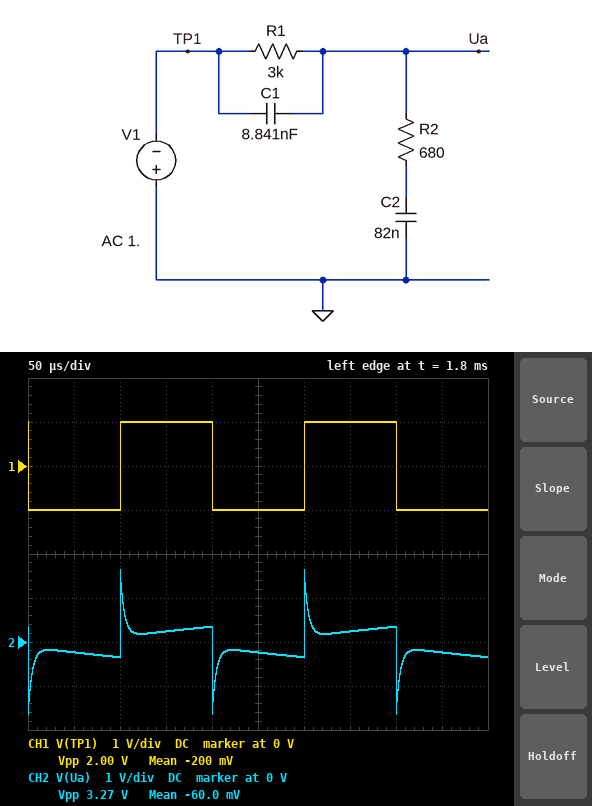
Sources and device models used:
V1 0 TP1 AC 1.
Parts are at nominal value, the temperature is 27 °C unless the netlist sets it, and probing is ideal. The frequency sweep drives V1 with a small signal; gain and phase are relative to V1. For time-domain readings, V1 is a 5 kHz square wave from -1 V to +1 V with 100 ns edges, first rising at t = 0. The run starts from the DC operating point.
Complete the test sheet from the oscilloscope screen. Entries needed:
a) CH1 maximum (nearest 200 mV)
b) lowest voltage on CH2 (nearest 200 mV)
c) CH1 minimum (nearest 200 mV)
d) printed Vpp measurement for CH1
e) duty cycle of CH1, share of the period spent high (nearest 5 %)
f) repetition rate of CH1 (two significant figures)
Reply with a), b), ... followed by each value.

a) 1.0 V
b) -1.6 V
c) -1.0 V
d) 2.00 V
e) 50 %
f) 5.0 kHz
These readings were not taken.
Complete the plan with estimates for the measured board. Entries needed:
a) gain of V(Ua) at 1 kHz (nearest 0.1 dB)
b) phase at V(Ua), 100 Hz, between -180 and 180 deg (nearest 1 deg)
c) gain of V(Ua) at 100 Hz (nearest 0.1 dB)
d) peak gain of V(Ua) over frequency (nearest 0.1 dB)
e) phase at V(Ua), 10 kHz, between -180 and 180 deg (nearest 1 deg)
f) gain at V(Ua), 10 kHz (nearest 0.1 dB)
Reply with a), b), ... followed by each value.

a) -6.5 dB
b) 171 deg
c) -0.2 dB
d) 0 dB
e) -150 deg
f) -9.5 dB
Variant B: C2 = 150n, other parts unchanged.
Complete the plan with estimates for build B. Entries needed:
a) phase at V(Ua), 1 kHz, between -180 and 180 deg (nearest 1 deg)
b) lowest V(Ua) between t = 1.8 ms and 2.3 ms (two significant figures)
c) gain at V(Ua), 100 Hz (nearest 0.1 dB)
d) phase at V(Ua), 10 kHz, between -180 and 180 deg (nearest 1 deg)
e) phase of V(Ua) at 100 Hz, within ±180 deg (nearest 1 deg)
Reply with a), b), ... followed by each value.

a) 146 deg
b) -1.7 V
c) -0.5 dB
d) -145 deg
e) 165 deg
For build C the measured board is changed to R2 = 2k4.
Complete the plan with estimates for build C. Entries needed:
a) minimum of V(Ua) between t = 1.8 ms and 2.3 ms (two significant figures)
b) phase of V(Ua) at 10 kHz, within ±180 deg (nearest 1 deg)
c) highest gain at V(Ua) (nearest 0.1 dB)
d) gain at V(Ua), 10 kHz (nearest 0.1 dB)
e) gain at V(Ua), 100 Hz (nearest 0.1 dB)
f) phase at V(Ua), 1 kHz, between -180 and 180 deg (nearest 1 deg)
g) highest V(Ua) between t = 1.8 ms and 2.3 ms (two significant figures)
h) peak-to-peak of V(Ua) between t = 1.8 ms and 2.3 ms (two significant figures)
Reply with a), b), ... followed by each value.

a) -1.5 V
b) -159 deg
c) 0 dB
d) -3.3 dB
e) -0.3 dB
f) 166 deg
g) 1.5 V
h) 3.0 V
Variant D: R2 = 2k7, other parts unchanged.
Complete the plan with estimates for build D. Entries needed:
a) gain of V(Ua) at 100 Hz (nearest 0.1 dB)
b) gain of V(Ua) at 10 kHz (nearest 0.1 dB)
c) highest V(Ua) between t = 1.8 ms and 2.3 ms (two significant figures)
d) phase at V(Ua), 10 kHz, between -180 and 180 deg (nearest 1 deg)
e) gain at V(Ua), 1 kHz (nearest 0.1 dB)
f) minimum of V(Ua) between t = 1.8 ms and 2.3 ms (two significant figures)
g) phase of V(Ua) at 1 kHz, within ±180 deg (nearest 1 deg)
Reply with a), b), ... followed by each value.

a) -0.3 dB
b) -3.0 dB
c) 1.5 V
d) -161 deg
e) -5.3 dB
f) -1.5 V
g) 168 deg
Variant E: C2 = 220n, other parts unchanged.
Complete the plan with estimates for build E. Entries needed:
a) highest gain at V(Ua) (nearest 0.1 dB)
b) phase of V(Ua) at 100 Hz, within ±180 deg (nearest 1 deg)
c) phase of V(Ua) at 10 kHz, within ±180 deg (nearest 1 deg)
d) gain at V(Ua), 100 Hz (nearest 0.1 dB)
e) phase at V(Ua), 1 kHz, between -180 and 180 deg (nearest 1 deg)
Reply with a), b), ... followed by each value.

a) 0 dB
b) 159 deg
c) -143 deg
d) -1.0 dB
e) 152 deg
